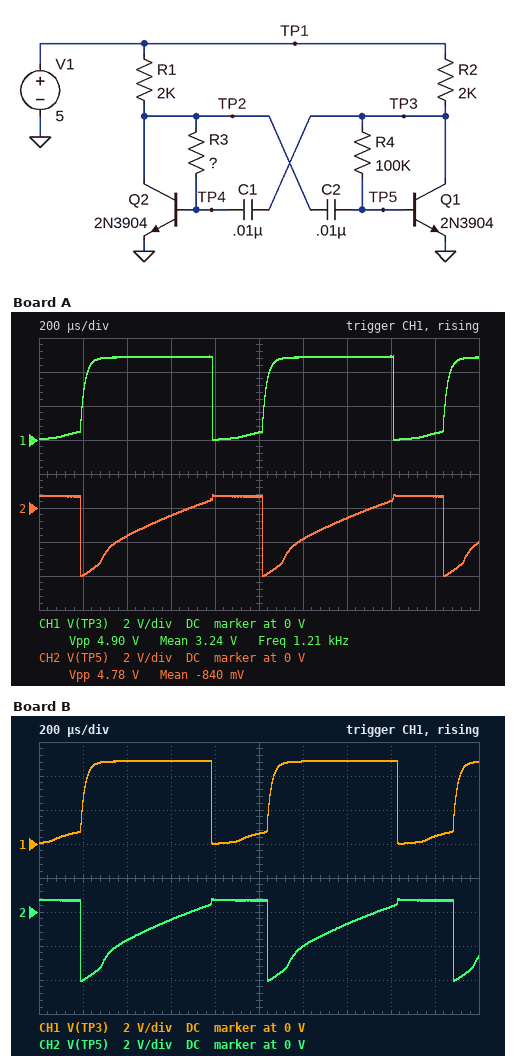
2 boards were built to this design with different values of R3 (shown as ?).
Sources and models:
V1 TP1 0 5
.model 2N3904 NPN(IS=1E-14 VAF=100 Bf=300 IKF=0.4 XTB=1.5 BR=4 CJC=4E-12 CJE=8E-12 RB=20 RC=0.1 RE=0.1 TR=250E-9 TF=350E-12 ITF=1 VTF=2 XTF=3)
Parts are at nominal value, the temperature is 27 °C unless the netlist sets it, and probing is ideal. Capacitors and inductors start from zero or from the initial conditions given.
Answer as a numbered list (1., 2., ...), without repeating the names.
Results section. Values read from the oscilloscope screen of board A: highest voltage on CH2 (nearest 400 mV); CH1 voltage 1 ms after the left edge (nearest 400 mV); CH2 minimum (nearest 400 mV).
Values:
1. 800 mV
2. 400 mV
3. -4.0 V
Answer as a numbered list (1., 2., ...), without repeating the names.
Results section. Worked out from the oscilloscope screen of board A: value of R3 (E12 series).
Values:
1. 33 kΩ
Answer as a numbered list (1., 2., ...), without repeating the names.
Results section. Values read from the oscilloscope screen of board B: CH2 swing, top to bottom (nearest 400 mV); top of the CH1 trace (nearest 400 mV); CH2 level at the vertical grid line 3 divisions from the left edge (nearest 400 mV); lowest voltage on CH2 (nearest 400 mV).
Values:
1. 4.8 V
2. 4.8 V
3. -400 mV
4. -4.0 V
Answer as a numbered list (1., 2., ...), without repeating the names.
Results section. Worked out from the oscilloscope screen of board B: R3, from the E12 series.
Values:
1. 39 kΩ
